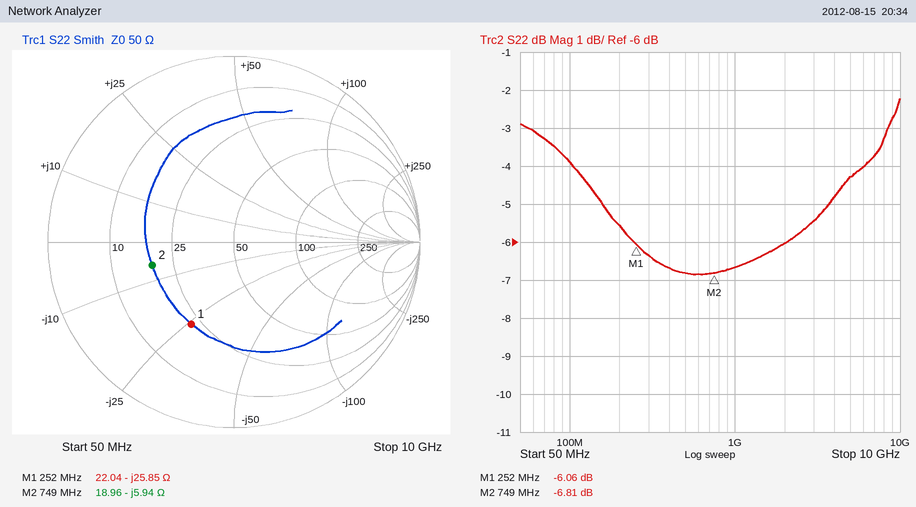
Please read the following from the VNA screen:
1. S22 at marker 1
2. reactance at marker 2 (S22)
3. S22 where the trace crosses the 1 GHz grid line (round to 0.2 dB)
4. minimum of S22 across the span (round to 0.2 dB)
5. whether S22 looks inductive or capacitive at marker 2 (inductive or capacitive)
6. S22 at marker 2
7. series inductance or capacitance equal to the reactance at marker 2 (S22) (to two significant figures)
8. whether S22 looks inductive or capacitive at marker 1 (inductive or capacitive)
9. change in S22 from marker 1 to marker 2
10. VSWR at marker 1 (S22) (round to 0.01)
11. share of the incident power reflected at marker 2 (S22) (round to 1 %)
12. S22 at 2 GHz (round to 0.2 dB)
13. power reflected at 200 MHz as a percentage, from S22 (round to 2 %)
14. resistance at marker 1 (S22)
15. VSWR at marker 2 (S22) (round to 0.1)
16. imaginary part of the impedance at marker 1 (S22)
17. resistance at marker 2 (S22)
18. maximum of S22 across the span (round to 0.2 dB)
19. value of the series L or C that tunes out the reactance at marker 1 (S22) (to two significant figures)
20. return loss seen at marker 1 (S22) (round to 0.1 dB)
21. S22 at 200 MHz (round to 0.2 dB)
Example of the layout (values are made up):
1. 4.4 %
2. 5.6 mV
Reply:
1. -6.06 dB
2. -5.94 Ω
3. -6.6 dB
4. -6.8 dB
5. capacitive
6. -6.81 dB
7. 36 pF
8. capacitive
9. -0.75 dB
10. 2.98
11. 21 %
12. -6.0 dB
13. 28 %
14. 22.04 Ω
15. 2.7
16. -25.85 Ω
17. 18.96 Ω
18. -2.2 dB
19. 16 nH
20. 6.1 dB
21. -5.6 dB
